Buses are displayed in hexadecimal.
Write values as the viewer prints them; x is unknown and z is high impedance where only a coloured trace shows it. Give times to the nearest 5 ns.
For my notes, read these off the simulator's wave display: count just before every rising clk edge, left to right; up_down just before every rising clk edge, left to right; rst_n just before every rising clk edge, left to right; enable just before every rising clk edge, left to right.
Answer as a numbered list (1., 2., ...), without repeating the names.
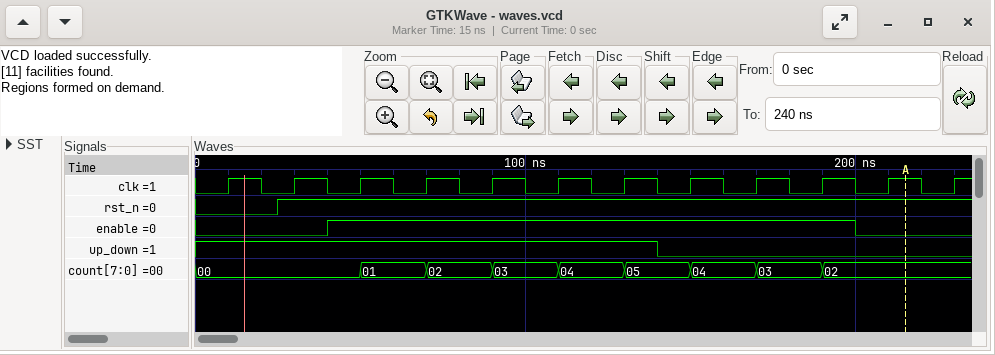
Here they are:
1. 00, 00, 00, 01, 02, 03, 04, 05, 04, 03, 02, 02
2. 1 1 1 1 1 1 1 0 0 0 0 0
3. 0 1 1 1 1 1 1 1 1 1 1 1
4. 0 0 1 1 1 1 1 1 1 1 0 0
